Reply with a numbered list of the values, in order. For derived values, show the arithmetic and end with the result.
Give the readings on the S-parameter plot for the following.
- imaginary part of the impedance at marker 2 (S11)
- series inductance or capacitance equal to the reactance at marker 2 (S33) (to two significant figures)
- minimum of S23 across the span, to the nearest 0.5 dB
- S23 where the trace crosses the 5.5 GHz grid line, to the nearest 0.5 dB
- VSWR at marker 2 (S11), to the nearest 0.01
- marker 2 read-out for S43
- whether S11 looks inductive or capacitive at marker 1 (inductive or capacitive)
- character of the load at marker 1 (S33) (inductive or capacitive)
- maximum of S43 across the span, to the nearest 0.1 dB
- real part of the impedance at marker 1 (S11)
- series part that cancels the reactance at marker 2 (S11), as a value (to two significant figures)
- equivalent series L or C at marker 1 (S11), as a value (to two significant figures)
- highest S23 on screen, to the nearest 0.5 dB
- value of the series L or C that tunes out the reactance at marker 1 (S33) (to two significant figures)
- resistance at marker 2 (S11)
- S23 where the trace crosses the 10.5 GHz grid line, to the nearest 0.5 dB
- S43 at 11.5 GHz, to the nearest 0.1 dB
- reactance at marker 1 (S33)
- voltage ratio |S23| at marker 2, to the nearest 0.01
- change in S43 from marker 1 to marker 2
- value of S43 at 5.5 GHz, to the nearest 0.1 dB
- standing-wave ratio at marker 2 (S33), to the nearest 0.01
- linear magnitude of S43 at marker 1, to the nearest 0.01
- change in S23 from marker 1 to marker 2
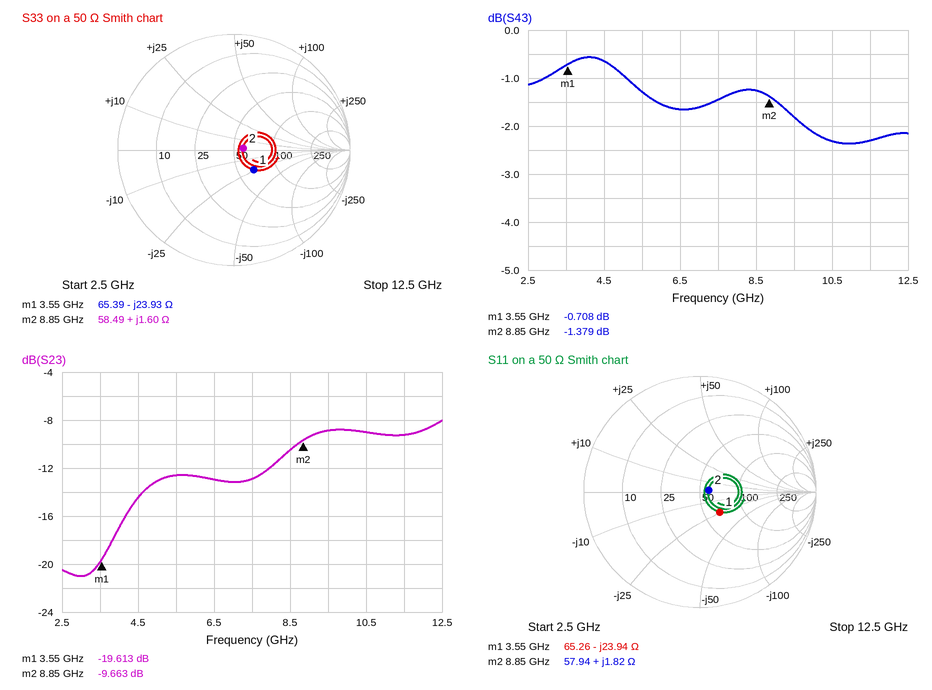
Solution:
1. +1.82 Ω
2. L = 1.6 Ω/(2π × 8.85 GHz) ≈ 29 pH
3. -21.0 dB
4. -12.5 dB
5. 1.16
6. -1.379 dB
7. capacitive
8. capacitive
9. -0.6 dB
10. 65.26 Ω
11. C = 1/(2π × 8.85 GHz × 1.82 Ω) ≈ 9.9 pF
12. C = 1/(2π × 3.55 GHz × 23.94 Ω) ≈ 1.9 pF
13. -8.0 dB
14. L = 23.93 Ω/(2π × 3.55 GHz) ≈ 1.1 nH
15. 57.94 Ω
16. -9.0 dB
17. -2.3 dB
18. -23.93 Ω
19. 10^(-9.663/20) ≈ 0.33
20. -1.379 − (-0.708) = -0.671 dB
21. -1.3 dB
22. 1.17
23. 10^(-0.708/20) ≈ 0.92
24. -9.663 − (-19.613) = 9.950 dB
